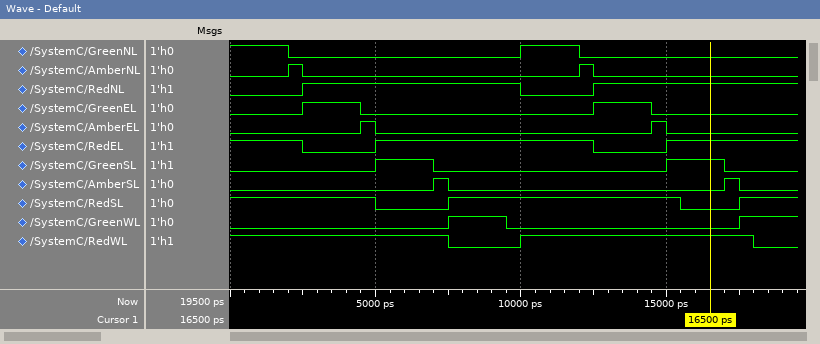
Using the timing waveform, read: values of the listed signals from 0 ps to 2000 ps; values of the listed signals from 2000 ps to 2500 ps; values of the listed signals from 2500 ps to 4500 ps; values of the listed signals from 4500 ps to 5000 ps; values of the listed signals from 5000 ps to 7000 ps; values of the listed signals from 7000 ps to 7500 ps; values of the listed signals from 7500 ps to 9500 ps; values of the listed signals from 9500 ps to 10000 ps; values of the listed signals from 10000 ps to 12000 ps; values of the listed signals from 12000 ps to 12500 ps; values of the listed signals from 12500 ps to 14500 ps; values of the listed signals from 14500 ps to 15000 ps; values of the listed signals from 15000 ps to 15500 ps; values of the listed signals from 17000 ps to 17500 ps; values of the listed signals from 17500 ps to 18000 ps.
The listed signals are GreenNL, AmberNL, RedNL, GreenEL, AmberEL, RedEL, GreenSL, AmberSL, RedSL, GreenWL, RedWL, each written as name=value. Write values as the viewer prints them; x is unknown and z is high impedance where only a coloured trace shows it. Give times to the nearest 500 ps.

GreenNL=1, AmberNL=0, RedNL=0, GreenEL=0, AmberEL=0, RedEL=1, GreenSL=0, AmberSL=0, RedSL=1, GreenWL=0, RedWL=1
GreenNL=0, AmberNL=1, RedNL=0, GreenEL=0, AmberEL=0, RedEL=1, GreenSL=0, AmberSL=0, RedSL=1, GreenWL=0, RedWL=1
GreenNL=0, AmberNL=0, RedNL=1, GreenEL=1, AmberEL=0, RedEL=0, GreenSL=0, AmberSL=0, RedSL=1, GreenWL=0, RedWL=1
GreenNL=0, AmberNL=0, RedNL=1, GreenEL=0, AmberEL=1, RedEL=0, GreenSL=0, AmberSL=0, RedSL=1, GreenWL=0, RedWL=1
GreenNL=0, AmberNL=0, RedNL=1, GreenEL=0, AmberEL=0, RedEL=1, GreenSL=1, AmberSL=0, RedSL=0, GreenWL=0, RedWL=1
GreenNL=0, AmberNL=0, RedNL=1, GreenEL=0, AmberEL=0, RedEL=1, GreenSL=0, AmberSL=1, RedSL=0, GreenWL=0, RedWL=1
GreenNL=0, AmberNL=0, RedNL=1, GreenEL=0, AmberEL=0, RedEL=1, GreenSL=0, AmberSL=0, RedSL=1, GreenWL=1, RedWL=0
GreenNL=0, AmberNL=0, RedNL=1, GreenEL=0, AmberEL=0, RedEL=1, GreenSL=0, AmberSL=0, RedSL=1, GreenWL=0, RedWL=0
GreenNL=1, AmberNL=0, RedNL=0, GreenEL=0, AmberEL=0, RedEL=1, GreenSL=0, AmberSL=0, RedSL=1, GreenWL=0, RedWL=1
GreenNL=0, AmberNL=1, RedNL=0, GreenEL=0, AmberEL=0, RedEL=1, GreenSL=0, AmberSL=0, RedSL=1, GreenWL=0, RedWL=1
GreenNL=0, AmberNL=0, RedNL=1, GreenEL=1, AmberEL=0, RedEL=0, GreenSL=0, AmberSL=0, RedSL=1, GreenWL=0, RedWL=1
GreenNL=0, AmberNL=0, RedNL=1, GreenEL=0, AmberEL=1, RedEL=0, GreenSL=0, AmberSL=0, RedSL=1, GreenWL=0, RedWL=1
GreenNL=0, AmberNL=0, RedNL=1, GreenEL=0, AmberEL=0, RedEL=1, GreenSL=1, AmberSL=0, RedSL=1, GreenWL=0, RedWL=1
GreenNL=0, AmberNL=0, RedNL=1, GreenEL=0, AmberEL=0, RedEL=1, GreenSL=0, AmberSL=1, RedSL=0, GreenWL=0, RedWL=1
GreenNL=0, AmberNL=0, RedNL=1, GreenEL=0, AmberEL=0, RedEL=1, GreenSL=0, AmberSL=0, RedSL=1, GreenWL=1, RedWL=1
